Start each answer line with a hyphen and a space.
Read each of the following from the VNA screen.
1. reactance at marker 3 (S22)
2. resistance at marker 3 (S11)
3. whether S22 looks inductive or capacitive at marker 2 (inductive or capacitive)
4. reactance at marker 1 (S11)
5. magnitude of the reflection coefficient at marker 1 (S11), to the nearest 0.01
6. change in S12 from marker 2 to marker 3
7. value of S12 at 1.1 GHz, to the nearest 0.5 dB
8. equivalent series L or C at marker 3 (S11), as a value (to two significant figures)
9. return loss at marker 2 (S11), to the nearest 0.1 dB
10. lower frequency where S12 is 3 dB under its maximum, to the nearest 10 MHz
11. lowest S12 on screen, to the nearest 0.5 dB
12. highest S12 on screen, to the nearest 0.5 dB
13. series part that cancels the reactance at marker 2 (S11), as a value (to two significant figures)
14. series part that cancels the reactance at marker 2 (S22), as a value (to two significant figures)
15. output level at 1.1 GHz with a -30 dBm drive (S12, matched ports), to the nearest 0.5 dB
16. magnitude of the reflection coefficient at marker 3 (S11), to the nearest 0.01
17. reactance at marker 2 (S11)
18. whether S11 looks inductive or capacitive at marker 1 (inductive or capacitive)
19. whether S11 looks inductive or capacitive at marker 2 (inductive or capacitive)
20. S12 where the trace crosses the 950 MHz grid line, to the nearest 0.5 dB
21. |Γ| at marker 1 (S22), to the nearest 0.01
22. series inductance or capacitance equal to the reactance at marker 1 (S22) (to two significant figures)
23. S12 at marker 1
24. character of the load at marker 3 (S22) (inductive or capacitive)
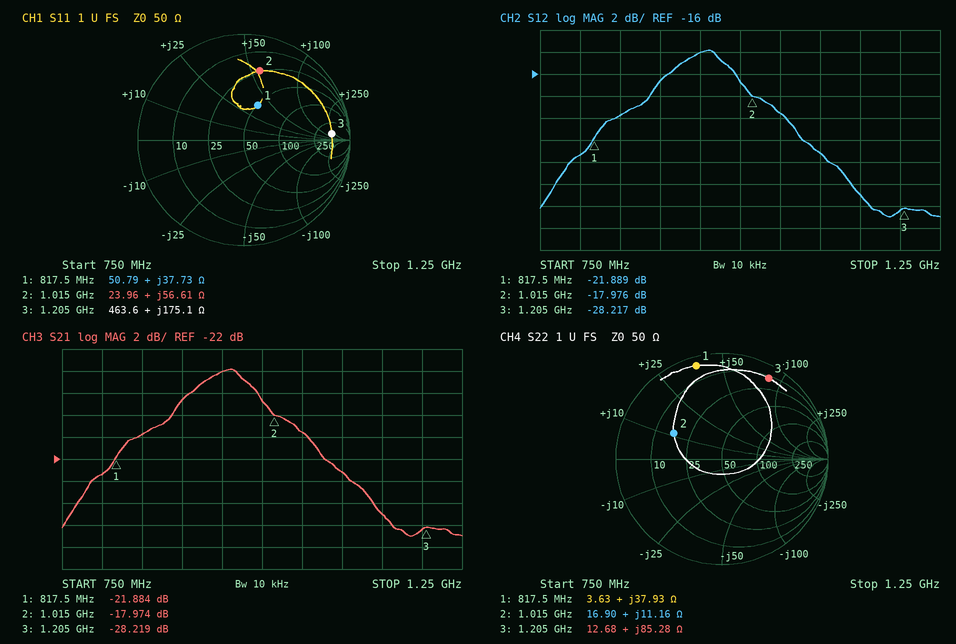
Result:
- +85.28 Ω
- 463.6 Ω
- inductive
- +37.73 Ω
- 0.35
- -10.241 dB
- -23.0 dB
- 23 nH
- 3.5 dB
- 900 MHz
- -29.0 dB
- -14.0 dB
- 2.8 pF
- 14 pF
- -53.0 dBm
- 0.83
- +56.61 Ω
- inductive
- inductive
- -14.0 dB
- 0.91
- 7.4 nH
- -21.889 dB
- inductive
